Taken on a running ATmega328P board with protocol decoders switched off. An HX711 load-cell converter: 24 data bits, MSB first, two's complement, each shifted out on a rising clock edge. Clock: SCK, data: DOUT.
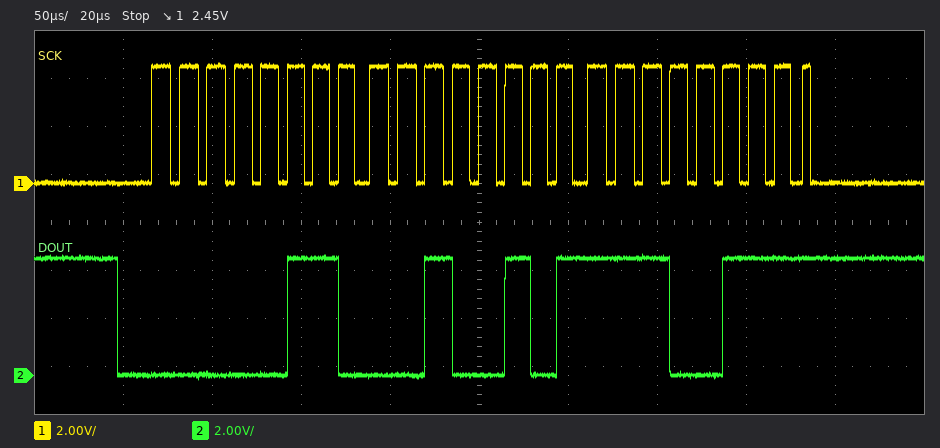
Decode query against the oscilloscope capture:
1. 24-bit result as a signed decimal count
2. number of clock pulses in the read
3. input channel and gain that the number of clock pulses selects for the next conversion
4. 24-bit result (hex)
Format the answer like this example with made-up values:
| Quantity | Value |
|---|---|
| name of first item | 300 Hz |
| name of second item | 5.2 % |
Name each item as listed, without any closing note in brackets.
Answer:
| Quantity | Value |
|---|---|
| 24-bit result as a signed decimal count | 402919 |
| number of clock pulses in the read | 25 |
| input channel and gain that the number of clock pulses selects for the next conversion | channel A, gain 128 |
| 24-bit result | 0x0625E7 |
